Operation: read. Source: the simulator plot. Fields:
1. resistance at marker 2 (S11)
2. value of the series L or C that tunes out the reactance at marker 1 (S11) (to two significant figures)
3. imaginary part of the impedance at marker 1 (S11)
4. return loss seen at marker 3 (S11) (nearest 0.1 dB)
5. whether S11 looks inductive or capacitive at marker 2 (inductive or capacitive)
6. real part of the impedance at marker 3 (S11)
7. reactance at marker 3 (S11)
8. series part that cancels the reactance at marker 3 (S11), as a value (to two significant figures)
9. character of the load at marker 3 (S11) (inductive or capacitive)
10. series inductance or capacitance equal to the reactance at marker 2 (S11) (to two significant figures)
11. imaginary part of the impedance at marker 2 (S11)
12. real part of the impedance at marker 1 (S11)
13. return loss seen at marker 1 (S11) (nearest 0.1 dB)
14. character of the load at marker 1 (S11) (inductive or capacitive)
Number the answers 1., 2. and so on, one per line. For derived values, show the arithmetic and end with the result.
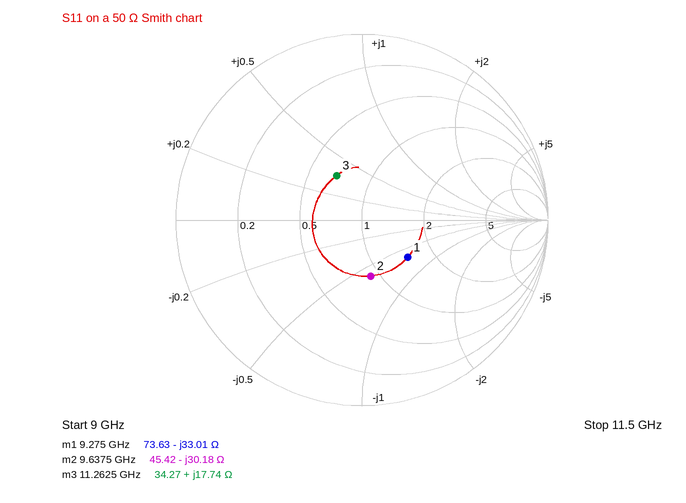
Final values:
1. 45.42 Ω
2. L = 33.01 Ω/(2π × 9.275 GHz) ≈ 566 pH, so 570 pH to two significant figures
3. -33.01 Ω
4. 11.2 dB
5. capacitive
6. 34.27 Ω
7. +17.74 Ω
8. C = 1/(2π × 11.2625 GHz × 17.74 Ω) ≈ 797 fF, so 800 fF to two significant figures
9. inductive
10. C = 1/(2π × 9.6375 GHz × 30.18 Ω) ≈ 547 fF, so 550 fF to two significant figures
11. -30.18 Ω
12. 73.63 Ω
13. 10.0 dB
14. capacitive
